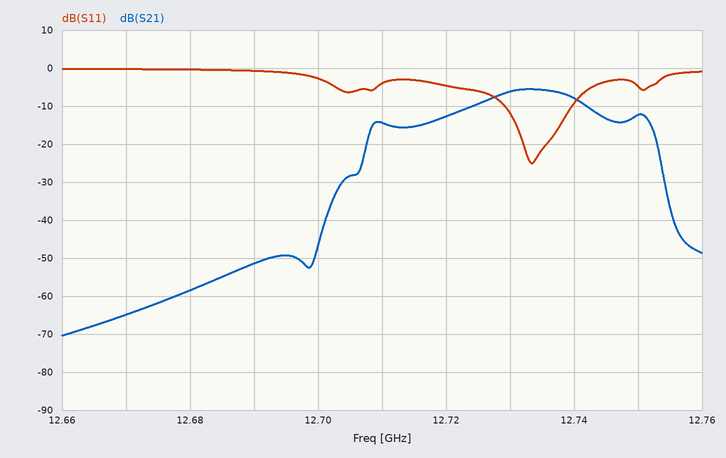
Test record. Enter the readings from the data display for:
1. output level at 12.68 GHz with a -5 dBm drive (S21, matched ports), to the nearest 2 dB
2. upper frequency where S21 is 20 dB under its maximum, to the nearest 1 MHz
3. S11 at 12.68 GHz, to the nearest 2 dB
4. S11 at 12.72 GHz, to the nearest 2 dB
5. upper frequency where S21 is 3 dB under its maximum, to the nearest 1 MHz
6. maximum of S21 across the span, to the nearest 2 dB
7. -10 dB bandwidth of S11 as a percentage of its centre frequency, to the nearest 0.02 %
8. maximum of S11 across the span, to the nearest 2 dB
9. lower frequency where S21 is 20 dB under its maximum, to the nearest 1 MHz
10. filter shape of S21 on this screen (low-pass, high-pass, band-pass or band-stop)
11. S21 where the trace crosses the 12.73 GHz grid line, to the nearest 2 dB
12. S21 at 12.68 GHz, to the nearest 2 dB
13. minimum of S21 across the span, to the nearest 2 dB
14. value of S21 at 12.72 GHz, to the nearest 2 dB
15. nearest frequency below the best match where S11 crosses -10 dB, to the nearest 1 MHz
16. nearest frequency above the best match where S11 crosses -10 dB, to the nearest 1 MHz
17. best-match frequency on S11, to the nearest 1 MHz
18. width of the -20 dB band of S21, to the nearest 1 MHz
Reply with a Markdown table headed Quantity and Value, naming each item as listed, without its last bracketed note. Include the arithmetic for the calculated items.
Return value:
| Quantity | Value |
|---|---|
| output level at 12.68 GHz with a -5 dBm drive (S21, matched ports), to the nearest 2 dB | -5 dBm + (-58 dB) = -64 dBm |
| upper frequency where S21 is 20 dB under its maximum, to the nearest 1 MHz | 12.754 GHz |
| S11 at 12.68 GHz, to the nearest 2 dB | 0 dB |
| S11 at 12.72 GHz, to the nearest 2 dB | -4 dB |
| upper frequency where S21 is 3 dB under its maximum, to the nearest 1 MHz | 12.741 GHz |
| maximum of S21 across the span, to the nearest 2 dB | -6 dB |
| -10 dB bandwidth of S11 as a percentage of its centre frequency, to the nearest 0.02 % | 11 MHz / 12.7345 GHz ≈ 0.0864 %, so 0.08 % to the nearest 0.02 % |
| maximum of S11 across the span, to the nearest 2 dB | 0 dB |
| lower frequency where S21 is 20 dB under its maximum, to the nearest 1 MHz | 12.707 GHz |
| filter shape of S21 on this screen | band-pass |
| S21 where the trace crosses the 12.73 GHz grid line, to the nearest 2 dB | -6 dB |
| S21 at 12.68 GHz, to the nearest 2 dB | -58 dB |
| minimum of S21 across the span, to the nearest 2 dB | -70 dB |
| value of S21 at 12.72 GHz, to the nearest 2 dB | -12 dB |
| nearest frequency below the best match where S11 crosses -10 dB, to the nearest 1 MHz | 12.729 GHz |
| nearest frequency above the best match where S11 crosses -10 dB, to the nearest 1 MHz | 12.740 GHz |
| best-match frequency on S11, to the nearest 1 MHz | 12.733 GHz |
| width of the -20 dB band of S21, to the nearest 1 MHz | 12.754 GHz − 12.707 GHz = 47 MHz |
